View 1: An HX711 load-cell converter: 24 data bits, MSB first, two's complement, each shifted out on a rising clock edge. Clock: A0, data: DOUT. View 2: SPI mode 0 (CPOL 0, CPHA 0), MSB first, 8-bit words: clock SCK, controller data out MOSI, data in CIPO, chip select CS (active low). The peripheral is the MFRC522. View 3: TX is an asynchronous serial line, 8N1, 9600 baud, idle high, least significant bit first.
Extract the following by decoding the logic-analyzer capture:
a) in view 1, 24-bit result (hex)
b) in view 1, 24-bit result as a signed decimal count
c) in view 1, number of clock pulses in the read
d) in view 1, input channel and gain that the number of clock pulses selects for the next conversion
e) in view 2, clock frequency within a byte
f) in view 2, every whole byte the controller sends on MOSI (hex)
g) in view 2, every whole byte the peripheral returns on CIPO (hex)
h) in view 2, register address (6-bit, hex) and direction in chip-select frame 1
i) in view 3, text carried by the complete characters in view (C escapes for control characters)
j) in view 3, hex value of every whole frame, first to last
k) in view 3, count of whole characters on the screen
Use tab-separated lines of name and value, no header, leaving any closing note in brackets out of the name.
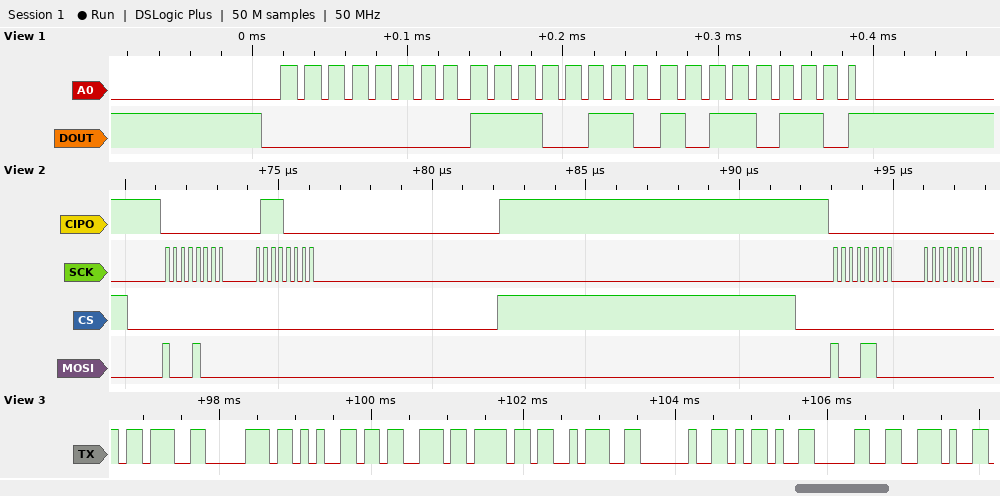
in view 1, 24-bit result	0x00E6B6
in view 1, 24-bit result as a signed decimal count	59062
in view 1, number of clock pulses in the read	25
in view 1, input channel and gain that the number of clock pulses selects for the next conversion	channel A, gain 128
in view 2, clock frequency within a byte	4 MHz
in view 2, every whole byte the controller sends on MOSI	88 00 8C 00
in view 2, every whole byte the peripheral returns on CIPO	00 70 00 00
in view 2, register address (6-bit, hex) and direction in chip-select frame 1	0x04 read
in view 3, text carried by the complete characters in view	";peso: -0."
in view 3, hex value of every whole frame, first to last	3B 70 65 73 6F 3A 20 2D 30 2E
in view 3, count of whole characters on the screen	10
